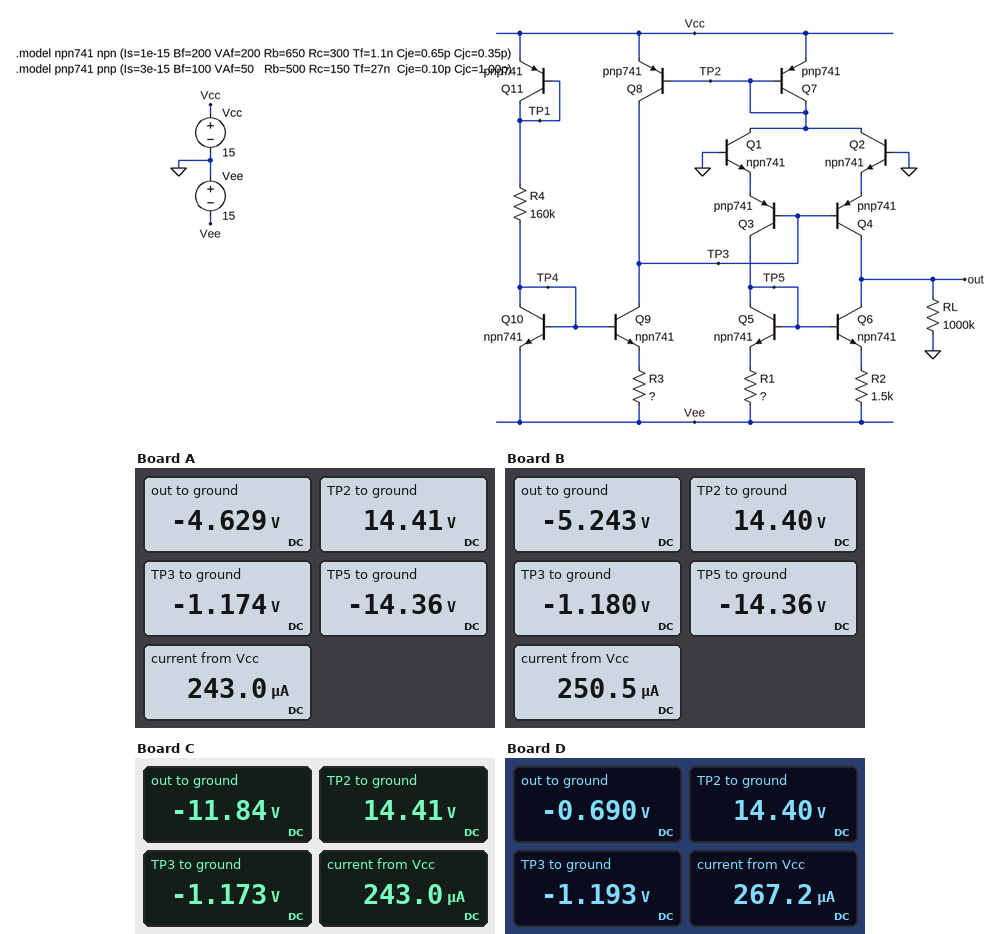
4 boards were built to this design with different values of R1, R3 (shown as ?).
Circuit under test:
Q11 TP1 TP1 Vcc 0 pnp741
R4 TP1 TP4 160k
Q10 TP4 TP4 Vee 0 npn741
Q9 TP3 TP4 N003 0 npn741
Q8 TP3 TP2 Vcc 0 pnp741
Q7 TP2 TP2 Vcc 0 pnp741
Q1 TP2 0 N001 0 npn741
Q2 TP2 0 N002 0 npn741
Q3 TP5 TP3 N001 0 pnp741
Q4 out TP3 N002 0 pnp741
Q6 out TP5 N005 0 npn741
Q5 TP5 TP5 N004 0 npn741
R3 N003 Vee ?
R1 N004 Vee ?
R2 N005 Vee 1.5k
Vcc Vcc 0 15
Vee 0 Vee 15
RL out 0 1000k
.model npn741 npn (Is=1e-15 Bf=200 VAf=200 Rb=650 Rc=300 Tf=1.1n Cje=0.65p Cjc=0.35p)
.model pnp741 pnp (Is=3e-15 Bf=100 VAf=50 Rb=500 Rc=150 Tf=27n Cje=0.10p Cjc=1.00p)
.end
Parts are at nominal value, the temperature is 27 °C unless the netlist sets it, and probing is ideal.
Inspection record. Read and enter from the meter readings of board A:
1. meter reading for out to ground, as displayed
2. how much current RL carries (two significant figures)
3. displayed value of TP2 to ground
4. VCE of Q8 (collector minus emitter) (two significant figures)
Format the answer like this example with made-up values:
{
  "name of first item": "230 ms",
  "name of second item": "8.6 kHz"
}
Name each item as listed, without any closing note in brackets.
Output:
{
  "meter reading for out to ground, as displayed": "-4.629 V",
  "how much current RL carries": "4.6 µA",
  "displayed value of TP2 to ground": "14.41 V",
  "VCE of Q8 (collector minus emitter)": "-16 V"
}
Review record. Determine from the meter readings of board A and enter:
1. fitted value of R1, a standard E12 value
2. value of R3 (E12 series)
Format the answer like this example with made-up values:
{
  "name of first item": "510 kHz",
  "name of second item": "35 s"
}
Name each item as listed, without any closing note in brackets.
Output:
{
  "fitted value of R1, a standard E12 value": "2.2 kΩ",
  "value of R3": "1.2 kΩ"
}
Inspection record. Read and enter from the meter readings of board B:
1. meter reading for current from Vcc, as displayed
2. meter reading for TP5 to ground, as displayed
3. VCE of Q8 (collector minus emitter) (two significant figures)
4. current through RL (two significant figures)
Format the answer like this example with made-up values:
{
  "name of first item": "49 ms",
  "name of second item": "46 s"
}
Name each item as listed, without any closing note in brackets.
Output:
{
  "meter reading for current from Vcc, as displayed": "250.5 µA",
  "meter reading for TP5 to ground, as displayed": "-14.36 V",
  "VCE of Q8 (collector minus emitter)": "-16 V",
  "current through RL": "5.2 µA"
}
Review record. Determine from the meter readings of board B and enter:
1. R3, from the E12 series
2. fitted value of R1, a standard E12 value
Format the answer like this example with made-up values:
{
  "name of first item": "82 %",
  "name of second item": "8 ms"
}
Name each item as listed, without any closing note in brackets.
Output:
{
  "R3, from the E12 series": "1 kΩ",
  "fitted value of R1, a standard E12 value": "2.2 kΩ"
}
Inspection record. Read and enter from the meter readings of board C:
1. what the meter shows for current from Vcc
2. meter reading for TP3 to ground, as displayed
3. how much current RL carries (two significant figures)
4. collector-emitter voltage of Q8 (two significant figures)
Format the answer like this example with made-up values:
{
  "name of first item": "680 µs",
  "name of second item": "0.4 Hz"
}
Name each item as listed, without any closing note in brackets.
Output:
{
  "what the meter shows for current from Vcc": "243.0 µA",
  "meter reading for TP3 to ground, as displayed": "-1.173 V",
  "how much current RL carries": "12 µA",
  "collector-emitter voltage of Q8": "-16 V"
}
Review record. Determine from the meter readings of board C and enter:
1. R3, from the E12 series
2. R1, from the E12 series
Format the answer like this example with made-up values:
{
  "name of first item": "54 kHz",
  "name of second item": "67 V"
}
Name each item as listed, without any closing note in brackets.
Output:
{
  "R3, from the E12 series": "1.2 kΩ",
  "R1, from the E12 series": "3.9 kΩ"
}
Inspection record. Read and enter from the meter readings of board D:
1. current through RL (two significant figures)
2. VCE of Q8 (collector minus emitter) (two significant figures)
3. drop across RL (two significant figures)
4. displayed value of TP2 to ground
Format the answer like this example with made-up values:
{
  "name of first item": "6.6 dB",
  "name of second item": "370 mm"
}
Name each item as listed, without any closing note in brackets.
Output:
{
  "current through RL": "690 nA",
  "VCE of Q8 (collector minus emitter)": "-16 V",
  "drop across RL": "690 mV",
  "displayed value of TP2 to ground": "14.40 V"
}
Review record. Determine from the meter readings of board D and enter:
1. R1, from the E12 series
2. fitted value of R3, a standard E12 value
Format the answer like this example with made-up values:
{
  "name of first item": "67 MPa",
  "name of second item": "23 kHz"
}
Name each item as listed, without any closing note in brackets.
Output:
{
  "R1, from the E12 series": "1 kΩ",
  "fitted value of R3, a standard E12 value": "680 Ω"
}
